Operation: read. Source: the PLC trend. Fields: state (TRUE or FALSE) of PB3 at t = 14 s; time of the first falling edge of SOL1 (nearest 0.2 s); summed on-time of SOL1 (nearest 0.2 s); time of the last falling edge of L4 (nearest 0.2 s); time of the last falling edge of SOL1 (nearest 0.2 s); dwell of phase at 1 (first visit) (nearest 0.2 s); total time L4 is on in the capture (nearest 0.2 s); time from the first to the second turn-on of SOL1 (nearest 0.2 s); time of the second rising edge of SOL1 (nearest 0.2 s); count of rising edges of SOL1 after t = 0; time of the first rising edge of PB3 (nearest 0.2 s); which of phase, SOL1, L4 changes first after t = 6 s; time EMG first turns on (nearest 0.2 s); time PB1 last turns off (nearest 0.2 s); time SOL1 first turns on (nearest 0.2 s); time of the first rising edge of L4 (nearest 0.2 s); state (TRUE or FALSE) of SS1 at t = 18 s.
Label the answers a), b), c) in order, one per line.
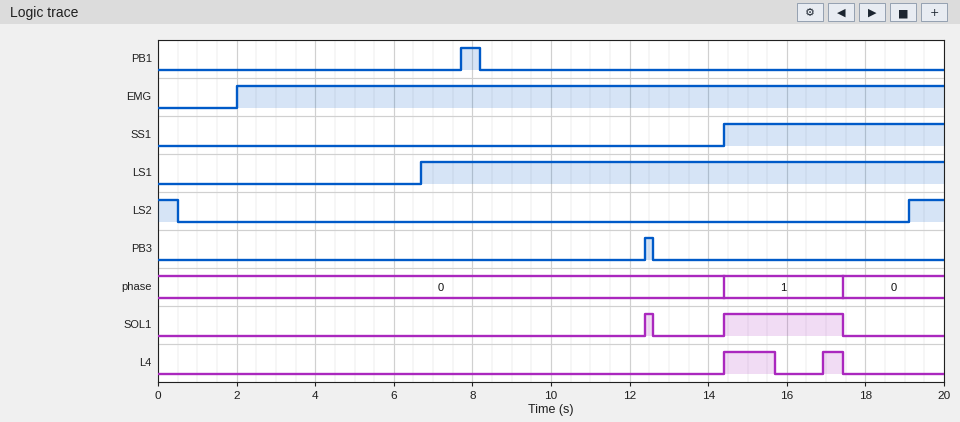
a) FALSE
b) 12.6 s
c) 3.2 s
d) 17.4 s
e) 17.4 s
f) 3.0 s
g) 1.8 s
h) 2.0 s
i) 14.4 s
j) 2
k) 12.4 s
l) SOL1
m) 2.0 s
n) 8.2 s
o) 12.4 s
p) 14.4 s
q) TRUE
